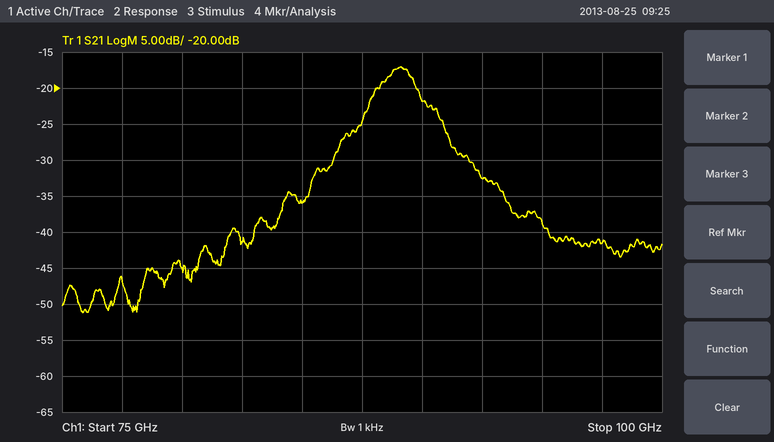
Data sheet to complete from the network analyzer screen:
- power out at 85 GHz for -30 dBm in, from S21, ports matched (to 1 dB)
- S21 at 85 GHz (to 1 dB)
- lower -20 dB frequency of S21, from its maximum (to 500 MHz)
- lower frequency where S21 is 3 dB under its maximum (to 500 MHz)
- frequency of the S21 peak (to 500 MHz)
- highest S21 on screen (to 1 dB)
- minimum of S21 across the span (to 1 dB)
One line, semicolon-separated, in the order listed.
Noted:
-66 dBm; -36 dB; 84.0 GHz; 88.0 GHz; 89.0 GHz; -17 dB; -51 dB
